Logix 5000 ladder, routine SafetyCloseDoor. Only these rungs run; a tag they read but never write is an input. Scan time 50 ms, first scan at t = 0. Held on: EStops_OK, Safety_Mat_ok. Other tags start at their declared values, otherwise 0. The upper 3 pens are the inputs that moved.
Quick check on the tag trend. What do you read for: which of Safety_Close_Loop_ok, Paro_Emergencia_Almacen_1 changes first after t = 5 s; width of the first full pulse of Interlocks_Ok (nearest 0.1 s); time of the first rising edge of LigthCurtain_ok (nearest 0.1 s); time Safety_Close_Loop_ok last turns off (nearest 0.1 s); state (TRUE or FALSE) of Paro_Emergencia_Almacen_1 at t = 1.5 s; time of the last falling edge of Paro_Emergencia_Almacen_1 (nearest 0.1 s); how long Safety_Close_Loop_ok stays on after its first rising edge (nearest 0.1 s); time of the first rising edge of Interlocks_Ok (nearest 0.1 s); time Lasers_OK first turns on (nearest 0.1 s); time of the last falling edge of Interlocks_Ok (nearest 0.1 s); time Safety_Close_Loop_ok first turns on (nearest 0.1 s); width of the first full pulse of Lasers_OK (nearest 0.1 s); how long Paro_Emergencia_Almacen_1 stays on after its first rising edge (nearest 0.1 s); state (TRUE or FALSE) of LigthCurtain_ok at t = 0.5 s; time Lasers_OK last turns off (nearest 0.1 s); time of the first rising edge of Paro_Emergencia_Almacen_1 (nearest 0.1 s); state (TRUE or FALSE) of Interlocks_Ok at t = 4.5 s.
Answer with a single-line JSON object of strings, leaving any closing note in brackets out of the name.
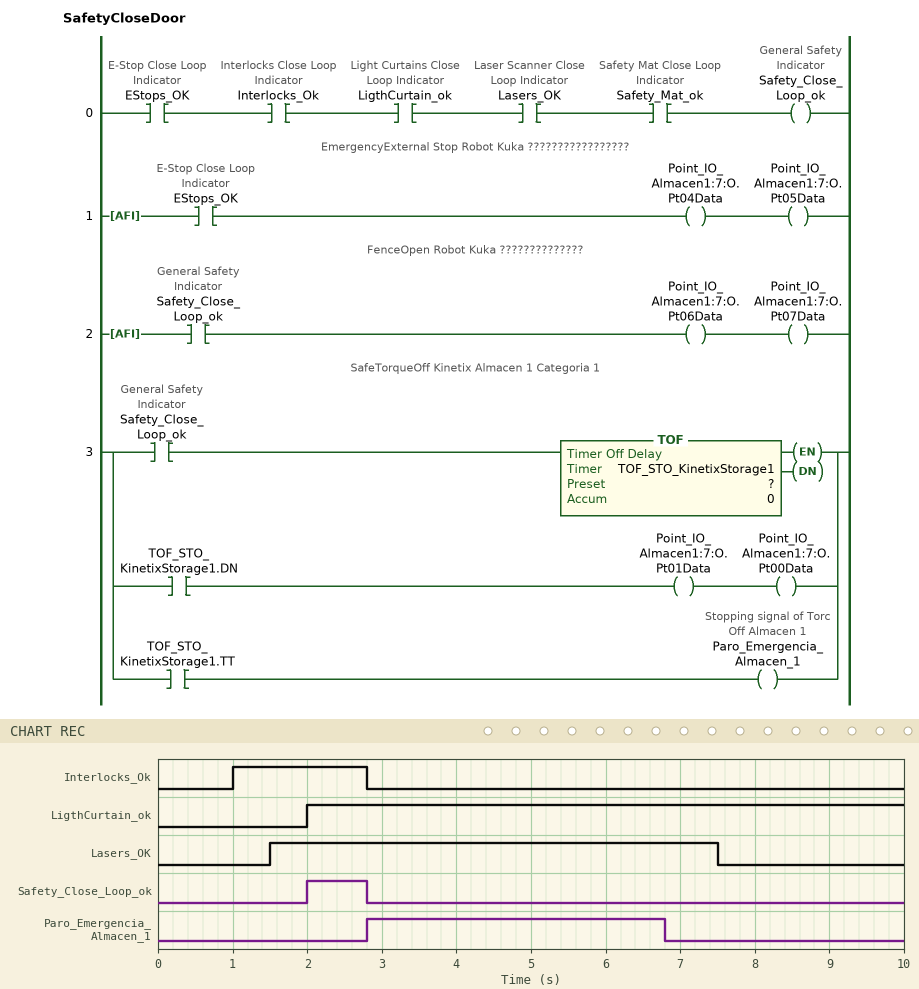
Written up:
{"which of Safety_Close_Loop_ok, Paro_Emergencia_Almacen_1 changes first after t = 5 s": "Paro_Emergencia_Almacen_1", "width of the first full pulse of Interlocks_Ok": "1.8 s", "time of the first rising edge of LigthCurtain_ok": "2.0 s", "time Safety_Close_Loop_ok last turns off": "2.8 s", "state (TRUE or FALSE) of Paro_Emergencia_Almacen_1 at t = 1.5 s": "FALSE", "time of the last falling edge of Paro_Emergencia_Almacen_1": "6.8 s", "how long Safety_Close_Loop_ok stays on after its first rising edge": "0.8 s", "time of the first rising edge of Interlocks_Ok": "1.0 s", "time Lasers_OK first turns on": "1.5 s", "time of the last falling edge of Interlocks_Ok": "2.8 s", "time Safety_Close_Loop_ok first turns on": "2.0 s", "width of the first full pulse of Lasers_OK": "6.0 s", "how long Paro_Emergencia_Almacen_1 stays on after its first rising edge": "4.0 s", "state (TRUE or FALSE) of LigthCurtain_ok at t = 0.5 s": "FALSE", "time Lasers_OK last turns off": "7.5 s", "time of the first rising edge of Paro_Emergencia_Almacen_1": "2.8 s", "state (TRUE or FALSE) of Interlocks_Ok at t = 4.5 s": "FALSE"}
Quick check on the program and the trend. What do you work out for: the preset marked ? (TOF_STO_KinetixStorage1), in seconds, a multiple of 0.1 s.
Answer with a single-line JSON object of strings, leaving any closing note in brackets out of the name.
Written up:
{"the preset marked ? (TOF_STO_KinetixStorage1), in seconds, a multiple of 0.1 s": "4.0 s"}
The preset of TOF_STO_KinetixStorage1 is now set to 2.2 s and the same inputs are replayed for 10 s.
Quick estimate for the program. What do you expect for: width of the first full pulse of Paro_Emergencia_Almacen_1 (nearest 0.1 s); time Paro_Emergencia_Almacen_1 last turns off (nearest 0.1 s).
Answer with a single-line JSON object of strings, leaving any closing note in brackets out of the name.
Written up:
{"width of the first full pulse of Paro_Emergencia_Almacen_1": "2.2 s", "time Paro_Emergencia_Almacen_1 last turns off": "5.0 s"}
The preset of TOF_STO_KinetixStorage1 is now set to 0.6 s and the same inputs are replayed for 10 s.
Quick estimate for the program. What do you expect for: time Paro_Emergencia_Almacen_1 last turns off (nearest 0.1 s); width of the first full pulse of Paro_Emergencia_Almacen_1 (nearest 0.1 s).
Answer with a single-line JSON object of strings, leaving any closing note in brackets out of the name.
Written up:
{"time Paro_Emergencia_Almacen_1 last turns off": "3.4 s", "width of the first full pulse of Paro_Emergencia_Almacen_1": "0.6 s"}
